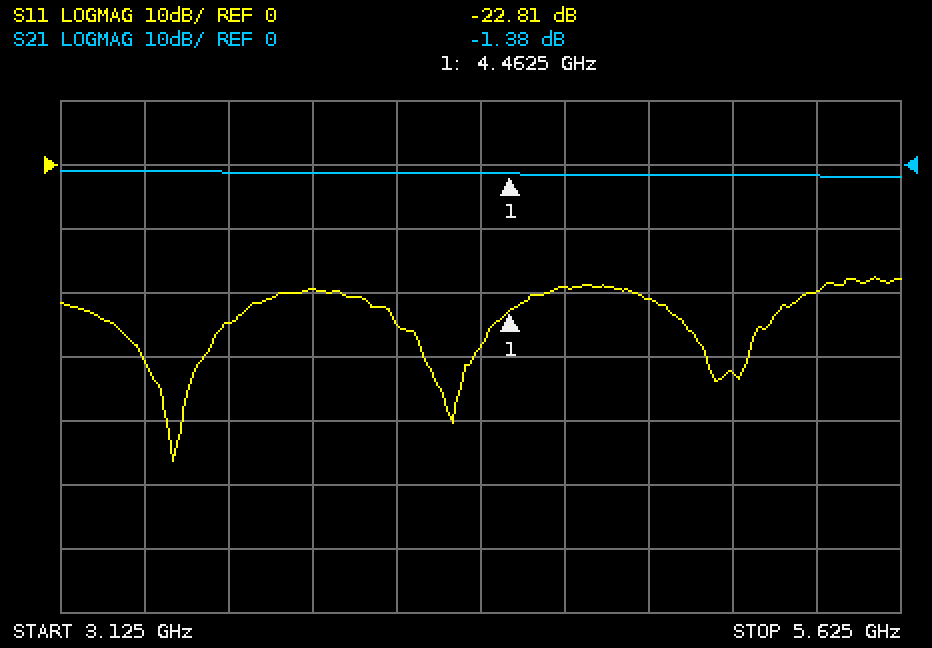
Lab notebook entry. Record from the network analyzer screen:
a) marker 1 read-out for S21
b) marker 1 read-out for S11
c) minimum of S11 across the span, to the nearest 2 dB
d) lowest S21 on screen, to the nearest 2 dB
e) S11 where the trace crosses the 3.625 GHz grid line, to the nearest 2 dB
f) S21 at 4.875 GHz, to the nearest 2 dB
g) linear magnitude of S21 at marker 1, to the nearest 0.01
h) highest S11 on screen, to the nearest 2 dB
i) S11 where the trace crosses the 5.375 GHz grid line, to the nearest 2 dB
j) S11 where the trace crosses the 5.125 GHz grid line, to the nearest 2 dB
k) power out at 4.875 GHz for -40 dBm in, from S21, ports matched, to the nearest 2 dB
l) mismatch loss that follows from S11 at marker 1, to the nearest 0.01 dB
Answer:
-1.38 dB
-22.81 dB
-46 dB
-2 dB
-24 dB
-2 dB
0.85
-18 dB
-20 dB
-32 dB
-42 dBm
0.02 dB
